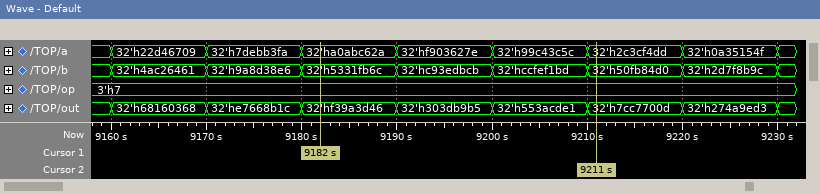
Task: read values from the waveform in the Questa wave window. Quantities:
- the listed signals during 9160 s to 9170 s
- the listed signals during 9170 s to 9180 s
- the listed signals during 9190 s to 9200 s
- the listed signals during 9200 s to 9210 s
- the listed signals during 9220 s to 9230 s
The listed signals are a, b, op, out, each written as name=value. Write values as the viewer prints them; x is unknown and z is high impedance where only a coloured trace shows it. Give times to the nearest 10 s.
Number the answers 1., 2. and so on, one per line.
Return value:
1. a=32'h22d46709, b=32'h4ac26461, op=3'h7, out=32'h68160368
2. a=32'h7debb3fa, b=32'h9a8d38e6, op=3'h7, out=32'he7668b1c
3. a=32'hf903627e, b=32'hc93edbcb, op=3'h7, out=32'h303db9b5
4. a=32'h99c43c5c, b=32'hccfef1bd, op=3'h7, out=32'h553acde1
5. a=32'h0a35154f, b=32'h2d7f8b9c, op=3'h7, out=32'h274a9ed3
